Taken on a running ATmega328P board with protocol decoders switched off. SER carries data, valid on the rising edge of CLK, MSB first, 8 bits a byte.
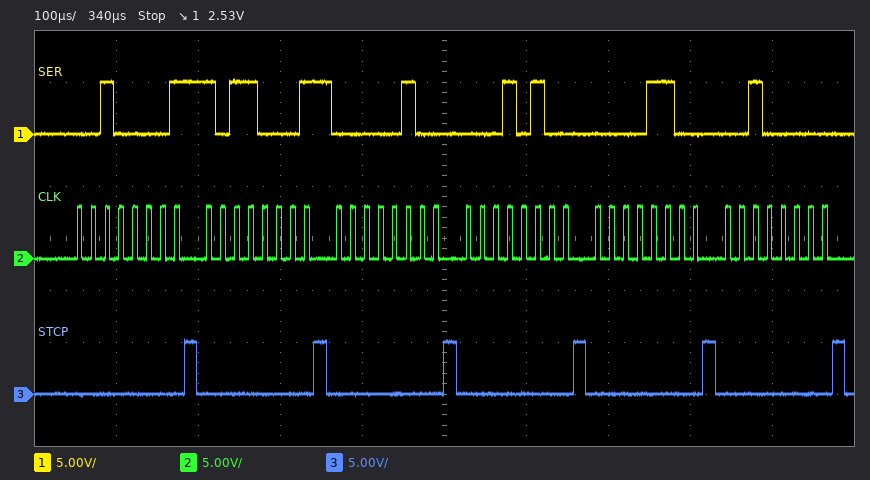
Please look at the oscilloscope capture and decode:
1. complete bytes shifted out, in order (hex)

0x21 0xB1 0x04 0x14 0x0C 0x20
